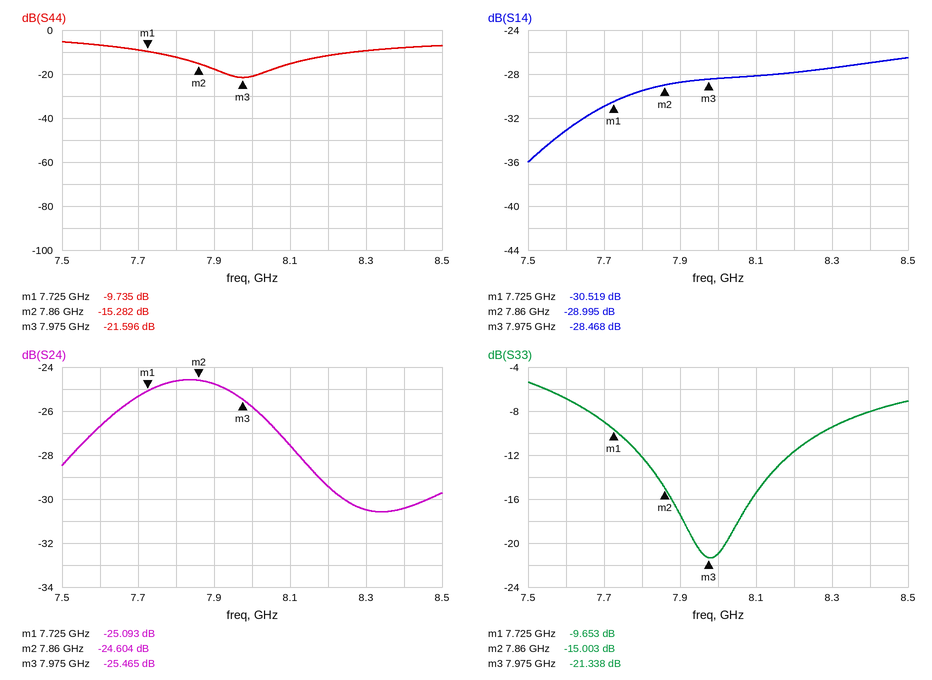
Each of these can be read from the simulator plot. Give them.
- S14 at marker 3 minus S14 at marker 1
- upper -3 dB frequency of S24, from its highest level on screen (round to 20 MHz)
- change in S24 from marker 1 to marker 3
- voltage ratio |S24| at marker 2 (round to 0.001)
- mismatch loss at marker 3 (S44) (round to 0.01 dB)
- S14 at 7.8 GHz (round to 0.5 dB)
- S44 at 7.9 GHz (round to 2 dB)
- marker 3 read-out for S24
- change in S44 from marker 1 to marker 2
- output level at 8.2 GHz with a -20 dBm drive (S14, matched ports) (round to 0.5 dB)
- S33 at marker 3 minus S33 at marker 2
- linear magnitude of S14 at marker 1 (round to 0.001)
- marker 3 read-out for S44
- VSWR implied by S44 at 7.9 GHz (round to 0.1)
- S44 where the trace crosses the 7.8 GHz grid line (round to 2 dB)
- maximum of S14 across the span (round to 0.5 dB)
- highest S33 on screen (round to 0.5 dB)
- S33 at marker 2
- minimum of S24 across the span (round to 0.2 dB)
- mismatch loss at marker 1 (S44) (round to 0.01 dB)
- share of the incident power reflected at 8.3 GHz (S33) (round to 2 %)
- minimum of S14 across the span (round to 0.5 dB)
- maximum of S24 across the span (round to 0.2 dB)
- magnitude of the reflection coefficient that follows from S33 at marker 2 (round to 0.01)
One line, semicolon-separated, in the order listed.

2.051 dB; 8.10 GHz; -0.372 dB; 0.059; 0.03 dB; -29.5 dB; -18 dB; -25.465 dB; -5.547 dB; -48.0 dBm; -6.335 dB; 0.030; -21.596 dB; 1.3; -12 dB; -26.5 dB; -5.5 dB; -15.003 dB; -30.6 dB; 0.49 dB; 12 %; -36.0 dB; -24.6 dB; 0.18
